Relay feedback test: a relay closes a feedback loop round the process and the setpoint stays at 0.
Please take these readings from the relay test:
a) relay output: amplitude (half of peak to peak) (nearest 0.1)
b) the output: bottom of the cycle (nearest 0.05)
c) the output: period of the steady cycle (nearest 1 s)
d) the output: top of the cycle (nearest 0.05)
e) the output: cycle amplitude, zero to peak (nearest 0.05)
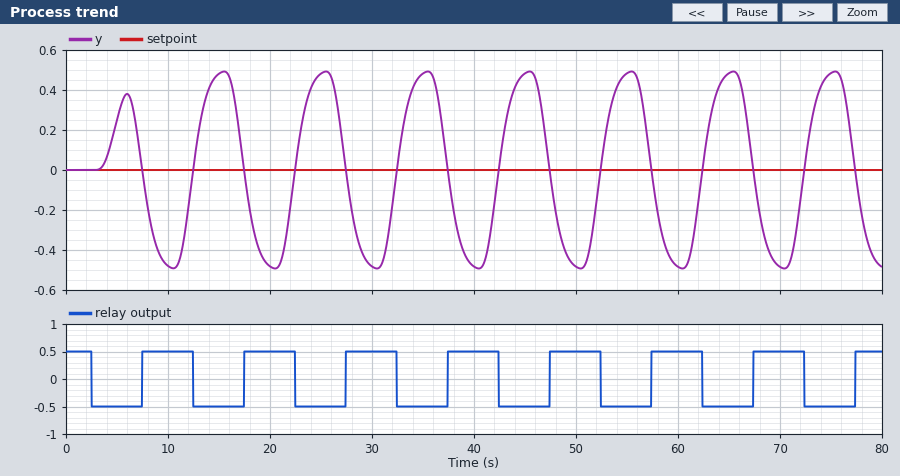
0.5
-0.50
10 s
0.50
0.50
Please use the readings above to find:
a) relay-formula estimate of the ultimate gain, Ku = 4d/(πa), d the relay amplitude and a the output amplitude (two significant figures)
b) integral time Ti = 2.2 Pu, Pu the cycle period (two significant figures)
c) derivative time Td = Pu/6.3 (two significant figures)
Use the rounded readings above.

1.3
22 s
1.6 s
